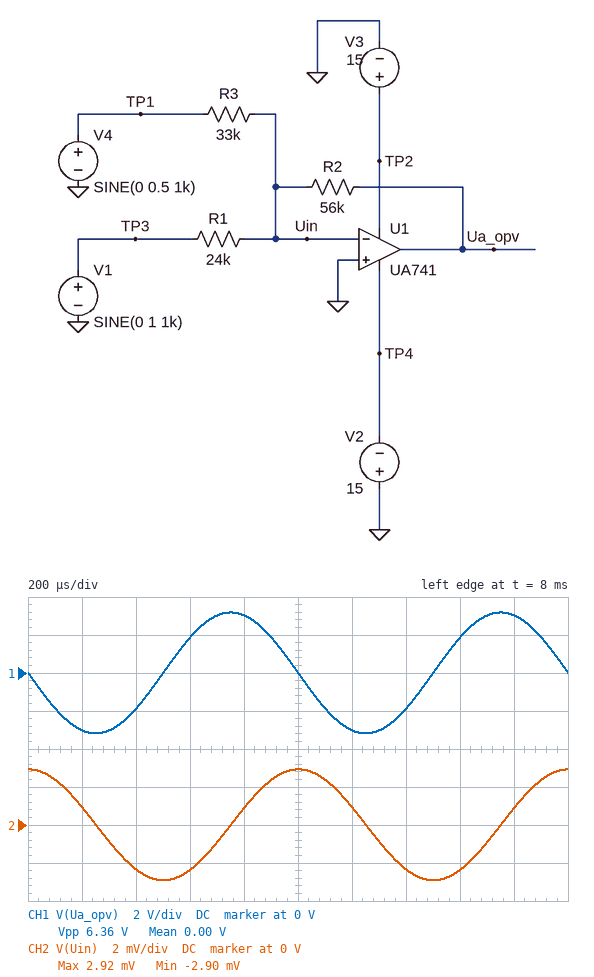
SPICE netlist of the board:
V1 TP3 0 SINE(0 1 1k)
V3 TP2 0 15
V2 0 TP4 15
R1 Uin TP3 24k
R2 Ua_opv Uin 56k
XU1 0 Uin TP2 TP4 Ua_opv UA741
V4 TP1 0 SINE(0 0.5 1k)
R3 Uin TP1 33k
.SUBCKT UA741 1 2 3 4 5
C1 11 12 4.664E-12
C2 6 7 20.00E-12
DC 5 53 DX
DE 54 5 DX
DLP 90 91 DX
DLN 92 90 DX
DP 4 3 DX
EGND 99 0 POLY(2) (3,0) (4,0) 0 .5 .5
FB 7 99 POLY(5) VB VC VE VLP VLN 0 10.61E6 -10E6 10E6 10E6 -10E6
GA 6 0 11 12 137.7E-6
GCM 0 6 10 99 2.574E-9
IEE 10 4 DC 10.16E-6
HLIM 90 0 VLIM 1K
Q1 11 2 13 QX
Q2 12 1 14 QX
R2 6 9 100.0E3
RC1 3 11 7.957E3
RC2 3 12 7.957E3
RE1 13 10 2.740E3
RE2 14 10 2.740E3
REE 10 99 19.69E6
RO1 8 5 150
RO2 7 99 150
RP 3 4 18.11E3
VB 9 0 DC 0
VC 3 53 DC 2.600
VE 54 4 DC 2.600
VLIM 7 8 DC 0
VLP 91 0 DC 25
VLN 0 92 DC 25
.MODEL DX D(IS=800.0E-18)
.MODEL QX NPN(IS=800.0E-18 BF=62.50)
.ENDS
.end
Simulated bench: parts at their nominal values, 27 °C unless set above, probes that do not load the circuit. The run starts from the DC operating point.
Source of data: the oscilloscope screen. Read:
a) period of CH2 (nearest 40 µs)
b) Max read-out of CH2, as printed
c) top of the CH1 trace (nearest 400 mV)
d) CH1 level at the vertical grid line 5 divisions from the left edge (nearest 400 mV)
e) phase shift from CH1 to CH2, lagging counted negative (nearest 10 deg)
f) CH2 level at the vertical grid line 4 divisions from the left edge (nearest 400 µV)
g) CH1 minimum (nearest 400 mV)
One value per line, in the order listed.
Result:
1.00 ms
2.92 mV
3.2 V
0 V
-90 deg
800 µV
-3.2 V
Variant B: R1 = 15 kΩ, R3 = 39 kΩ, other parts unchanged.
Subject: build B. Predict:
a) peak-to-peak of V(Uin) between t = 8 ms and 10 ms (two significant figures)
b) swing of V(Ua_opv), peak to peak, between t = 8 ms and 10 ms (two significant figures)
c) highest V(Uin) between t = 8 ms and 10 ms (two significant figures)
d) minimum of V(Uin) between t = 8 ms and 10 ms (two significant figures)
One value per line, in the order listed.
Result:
8.2 mV
8.9 V
4.1 mV
-4.1 mV
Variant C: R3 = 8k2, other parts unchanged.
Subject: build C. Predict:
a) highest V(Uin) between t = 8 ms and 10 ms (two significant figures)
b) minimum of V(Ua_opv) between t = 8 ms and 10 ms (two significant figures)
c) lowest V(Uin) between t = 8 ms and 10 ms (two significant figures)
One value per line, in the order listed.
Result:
5.3 mV
-5.7 V
-5.3 mV
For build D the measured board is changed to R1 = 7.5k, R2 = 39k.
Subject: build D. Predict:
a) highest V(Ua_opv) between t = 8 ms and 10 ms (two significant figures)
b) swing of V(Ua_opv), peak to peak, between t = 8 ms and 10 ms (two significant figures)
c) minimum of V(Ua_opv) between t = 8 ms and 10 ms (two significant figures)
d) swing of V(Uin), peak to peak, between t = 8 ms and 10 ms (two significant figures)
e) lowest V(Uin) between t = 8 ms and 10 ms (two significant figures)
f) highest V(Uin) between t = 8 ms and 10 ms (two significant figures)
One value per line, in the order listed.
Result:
5.8 V
12 V
-5.8 V
11 mV
-5.3 mV
5.3 mV
